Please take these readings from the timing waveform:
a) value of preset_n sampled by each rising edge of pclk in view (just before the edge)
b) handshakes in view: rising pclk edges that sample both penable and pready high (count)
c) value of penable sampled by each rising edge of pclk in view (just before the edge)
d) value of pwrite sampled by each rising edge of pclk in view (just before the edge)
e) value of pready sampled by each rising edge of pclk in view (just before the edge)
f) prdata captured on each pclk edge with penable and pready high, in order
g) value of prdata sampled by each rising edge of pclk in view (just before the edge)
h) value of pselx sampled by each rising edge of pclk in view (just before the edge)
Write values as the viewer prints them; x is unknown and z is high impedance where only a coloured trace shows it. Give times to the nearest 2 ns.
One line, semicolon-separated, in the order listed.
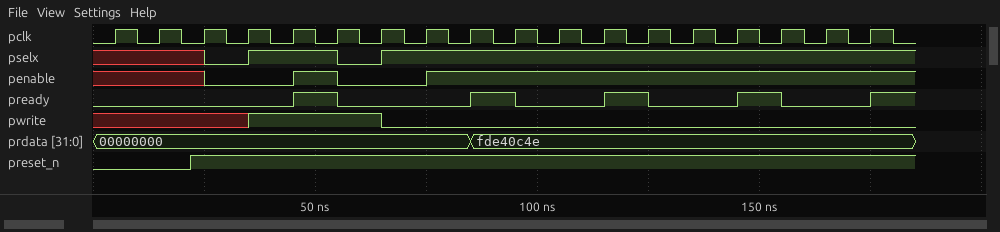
0 0 1 1 1 1 1 1 1 1 1 1 1 1 1 1 1 1; 4; x x x 0 0 1 0 0 1 1 1 1 1 1 1 1 1 1; x x x x 1 1 1 0 0 0 0 0 0 0 0 0 0 0; 0 0 0 0 0 1 0 0 0 1 0 0 1 0 0 1 0 0; 00000000, fde40c4e, fde40c4e, fde40c4e; 00000000, 00000000, 00000000, 00000000, 00000000, 00000000, 00000000, 00000000, 00000000, fde40c4e, fde40c4e, fde40c4e, fde40c4e, fde40c4e, fde40c4e, fde40c4e, fde40c4e, fde40c4e; x x x 0 1 1 0 1 1 1 1 1 1 1 1 1 1 1
